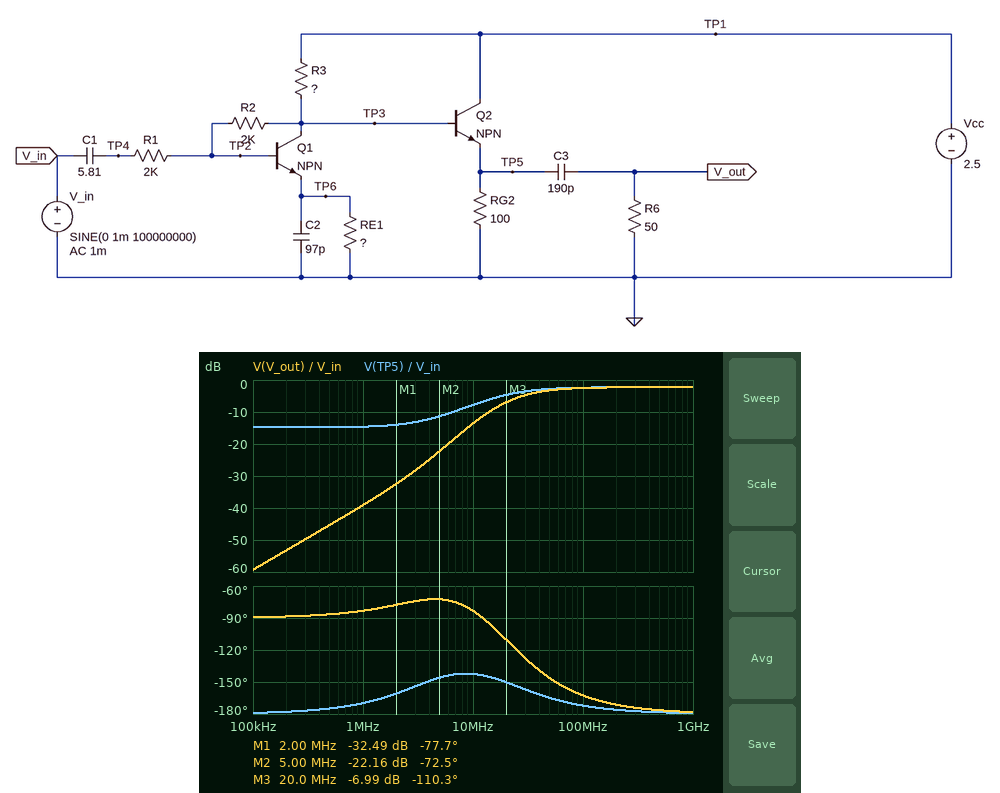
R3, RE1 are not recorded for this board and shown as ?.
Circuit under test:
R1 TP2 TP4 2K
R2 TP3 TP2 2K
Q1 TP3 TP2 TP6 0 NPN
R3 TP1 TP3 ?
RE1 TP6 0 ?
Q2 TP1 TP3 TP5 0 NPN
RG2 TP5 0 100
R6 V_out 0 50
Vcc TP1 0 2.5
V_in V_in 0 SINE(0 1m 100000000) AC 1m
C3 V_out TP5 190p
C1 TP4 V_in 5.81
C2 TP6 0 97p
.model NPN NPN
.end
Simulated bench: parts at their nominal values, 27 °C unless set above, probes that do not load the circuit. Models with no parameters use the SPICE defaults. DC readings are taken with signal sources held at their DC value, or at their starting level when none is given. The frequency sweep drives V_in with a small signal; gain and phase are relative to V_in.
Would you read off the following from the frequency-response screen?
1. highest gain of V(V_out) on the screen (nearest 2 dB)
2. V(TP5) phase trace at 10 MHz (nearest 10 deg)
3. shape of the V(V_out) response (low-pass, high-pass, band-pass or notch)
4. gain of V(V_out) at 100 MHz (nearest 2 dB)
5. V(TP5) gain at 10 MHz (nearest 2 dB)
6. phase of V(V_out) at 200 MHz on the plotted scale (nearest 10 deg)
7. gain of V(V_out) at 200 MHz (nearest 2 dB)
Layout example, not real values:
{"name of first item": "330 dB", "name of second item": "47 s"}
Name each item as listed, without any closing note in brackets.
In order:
{"highest gain of V(V_out) on the screen": "-2 dB", "V(TP5) phase trace at 10 MHz": "-140 deg", "shape of the V(V_out) response": "high-pass", "gain of V(V_out) at 100 MHz": "-2 dB", "V(TP5) gain at 10 MHz": "-8 dB", "phase of V(V_out) at 200 MHz on the plotted scale": "-170 deg", "gain of V(V_out) at 200 MHz": "-2 dB"}
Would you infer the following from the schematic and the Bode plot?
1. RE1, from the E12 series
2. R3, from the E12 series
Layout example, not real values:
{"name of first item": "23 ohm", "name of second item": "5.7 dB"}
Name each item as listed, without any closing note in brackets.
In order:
{"RE1, from the E12 series": "330 Ω", "R3, from the E12 series": "220 Ω"}
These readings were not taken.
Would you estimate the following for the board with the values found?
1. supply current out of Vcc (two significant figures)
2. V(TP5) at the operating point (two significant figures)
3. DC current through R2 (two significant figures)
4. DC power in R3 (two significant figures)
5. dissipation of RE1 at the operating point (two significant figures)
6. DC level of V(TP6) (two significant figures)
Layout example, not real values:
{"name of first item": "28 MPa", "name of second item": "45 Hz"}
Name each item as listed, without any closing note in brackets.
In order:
{"supply current out of Vcc": "13 mA", "V(TP5) at the operating point": "1.0 V", "DC current through R2": "29 µA", "DC power in R3": "2.0 mW", "dissipation of RE1 at the operating point": "2.9 mW", "DC level of V(TP6)": "970 mV"}
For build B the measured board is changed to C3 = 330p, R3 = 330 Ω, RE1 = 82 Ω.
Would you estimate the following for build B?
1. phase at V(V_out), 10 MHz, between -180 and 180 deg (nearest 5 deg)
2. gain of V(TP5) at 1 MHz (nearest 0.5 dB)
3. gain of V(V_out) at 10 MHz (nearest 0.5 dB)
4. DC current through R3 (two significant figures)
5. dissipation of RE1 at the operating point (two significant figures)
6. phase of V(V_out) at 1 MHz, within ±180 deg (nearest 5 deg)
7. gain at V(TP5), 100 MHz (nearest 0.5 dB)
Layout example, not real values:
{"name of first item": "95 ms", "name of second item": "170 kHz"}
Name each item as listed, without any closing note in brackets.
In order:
{"phase at V(V_out), 10 MHz, between -180 and 180 deg": "-130 deg", "gain of V(TP5) at 1 MHz": "-5.5 dB", "gain of V(V_out) at 10 MHz": "-8.5 dB", "DC current through R3": "3.9 mA", "dissipation of RE1 at the operating point": "1.2 mW", "phase of V(V_out) at 1 MHz, within ±180 deg": "-95 deg", "gain at V(TP5), 100 MHz": "-3.0 dB"}
